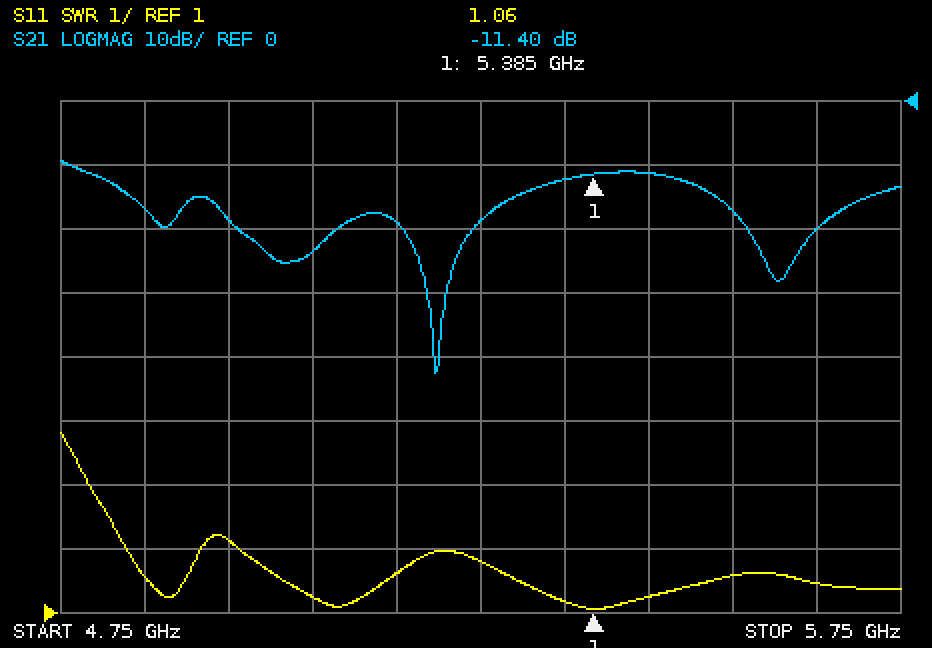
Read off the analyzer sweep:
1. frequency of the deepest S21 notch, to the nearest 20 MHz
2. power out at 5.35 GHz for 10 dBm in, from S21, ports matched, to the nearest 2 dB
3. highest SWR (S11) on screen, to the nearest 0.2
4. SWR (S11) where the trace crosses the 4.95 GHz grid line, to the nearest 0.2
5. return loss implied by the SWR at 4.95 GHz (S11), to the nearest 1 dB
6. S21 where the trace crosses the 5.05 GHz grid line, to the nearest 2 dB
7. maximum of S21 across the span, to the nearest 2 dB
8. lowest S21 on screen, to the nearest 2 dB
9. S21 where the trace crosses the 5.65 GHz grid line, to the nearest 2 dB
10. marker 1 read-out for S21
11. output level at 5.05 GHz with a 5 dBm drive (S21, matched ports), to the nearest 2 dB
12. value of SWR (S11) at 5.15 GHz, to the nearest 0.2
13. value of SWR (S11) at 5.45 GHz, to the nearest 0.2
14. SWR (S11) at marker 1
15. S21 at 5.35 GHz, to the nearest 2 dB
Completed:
5.20 GHz
-2 dBm
3.8
2.2
9 dB
-24 dB
-10 dB
-42 dB
-20 dB
-11.40 dB
-18 dBm
1.6
1.2
1.06
-12 dB
